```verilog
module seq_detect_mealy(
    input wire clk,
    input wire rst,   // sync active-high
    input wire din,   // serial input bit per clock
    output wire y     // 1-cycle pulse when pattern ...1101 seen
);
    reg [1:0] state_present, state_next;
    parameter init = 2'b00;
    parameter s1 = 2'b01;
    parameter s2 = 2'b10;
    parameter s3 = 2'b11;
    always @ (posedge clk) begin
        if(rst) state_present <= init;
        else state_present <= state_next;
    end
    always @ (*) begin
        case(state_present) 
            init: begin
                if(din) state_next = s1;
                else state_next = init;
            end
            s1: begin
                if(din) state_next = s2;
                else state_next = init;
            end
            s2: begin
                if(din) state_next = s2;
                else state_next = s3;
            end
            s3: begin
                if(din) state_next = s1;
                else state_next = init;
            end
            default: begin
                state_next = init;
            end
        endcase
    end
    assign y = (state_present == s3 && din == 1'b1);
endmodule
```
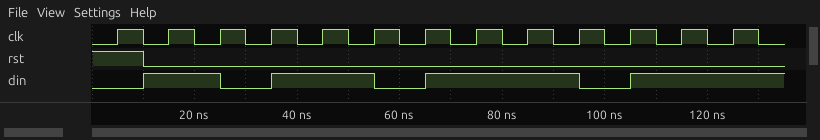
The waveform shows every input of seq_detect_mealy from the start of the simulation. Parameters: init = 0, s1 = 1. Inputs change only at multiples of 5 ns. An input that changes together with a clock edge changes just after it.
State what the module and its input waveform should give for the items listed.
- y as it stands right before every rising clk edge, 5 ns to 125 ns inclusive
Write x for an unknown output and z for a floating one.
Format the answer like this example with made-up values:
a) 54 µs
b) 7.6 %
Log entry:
a) 0 0 0 0 1 0 0 1 0 0 0 1 0
